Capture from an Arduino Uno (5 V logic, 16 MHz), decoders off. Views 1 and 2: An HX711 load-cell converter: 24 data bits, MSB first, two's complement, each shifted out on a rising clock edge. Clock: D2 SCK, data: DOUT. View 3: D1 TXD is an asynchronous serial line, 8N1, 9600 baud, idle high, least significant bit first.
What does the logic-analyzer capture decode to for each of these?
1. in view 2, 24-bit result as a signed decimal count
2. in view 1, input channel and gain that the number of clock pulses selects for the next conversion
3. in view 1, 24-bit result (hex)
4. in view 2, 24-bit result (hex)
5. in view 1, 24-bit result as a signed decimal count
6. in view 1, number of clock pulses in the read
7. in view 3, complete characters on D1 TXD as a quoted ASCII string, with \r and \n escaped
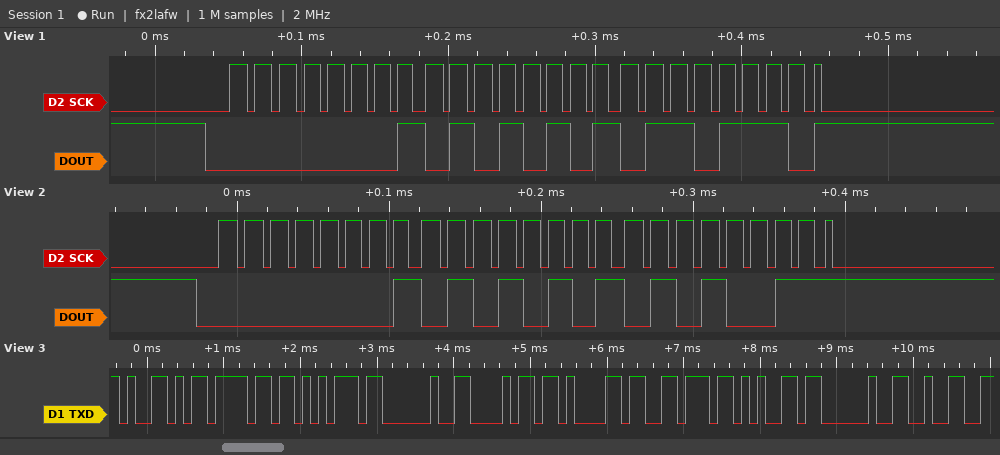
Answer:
87379
channel A, gain 128
0x01556E
0x015553
87406
25
"You have 2"
